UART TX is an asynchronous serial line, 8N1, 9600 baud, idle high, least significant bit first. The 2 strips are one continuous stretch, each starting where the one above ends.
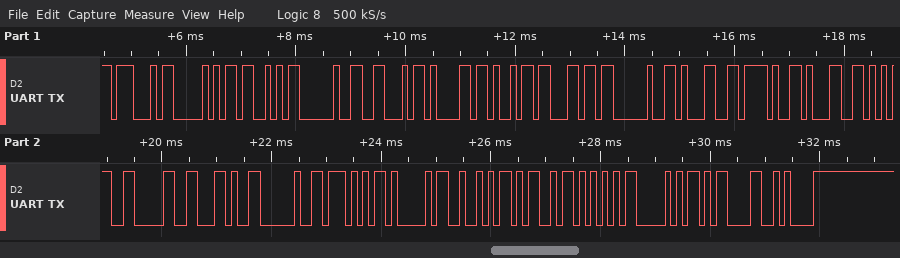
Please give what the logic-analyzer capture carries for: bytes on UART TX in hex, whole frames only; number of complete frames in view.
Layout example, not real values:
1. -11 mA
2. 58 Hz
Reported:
1. 47 50 53 20 46 61 69 6C 20 31 2F 31 35 30 2C 20 57 41 52 4D 55 50 0D 0A
2. 24
